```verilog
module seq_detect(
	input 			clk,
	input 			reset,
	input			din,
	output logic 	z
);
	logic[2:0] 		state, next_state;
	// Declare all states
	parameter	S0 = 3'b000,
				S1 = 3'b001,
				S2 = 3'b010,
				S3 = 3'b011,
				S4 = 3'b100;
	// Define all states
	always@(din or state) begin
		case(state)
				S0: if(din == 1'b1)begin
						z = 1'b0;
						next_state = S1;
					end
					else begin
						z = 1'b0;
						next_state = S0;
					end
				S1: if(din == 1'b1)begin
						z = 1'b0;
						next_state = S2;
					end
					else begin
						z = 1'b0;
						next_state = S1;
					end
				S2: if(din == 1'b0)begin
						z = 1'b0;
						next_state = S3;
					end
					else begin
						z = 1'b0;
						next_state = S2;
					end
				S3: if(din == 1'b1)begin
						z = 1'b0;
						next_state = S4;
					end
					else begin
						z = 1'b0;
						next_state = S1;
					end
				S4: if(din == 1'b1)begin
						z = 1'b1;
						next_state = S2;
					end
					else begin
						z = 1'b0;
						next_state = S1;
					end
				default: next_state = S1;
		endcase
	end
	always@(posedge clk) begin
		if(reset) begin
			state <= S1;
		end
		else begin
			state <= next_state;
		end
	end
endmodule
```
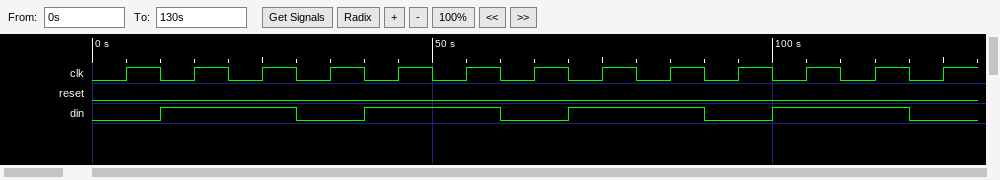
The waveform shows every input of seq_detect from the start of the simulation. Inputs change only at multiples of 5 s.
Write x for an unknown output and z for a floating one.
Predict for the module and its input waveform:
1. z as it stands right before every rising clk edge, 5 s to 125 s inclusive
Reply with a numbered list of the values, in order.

1. x 0 0 0 0 1 0 0 1 0 0 1 0
